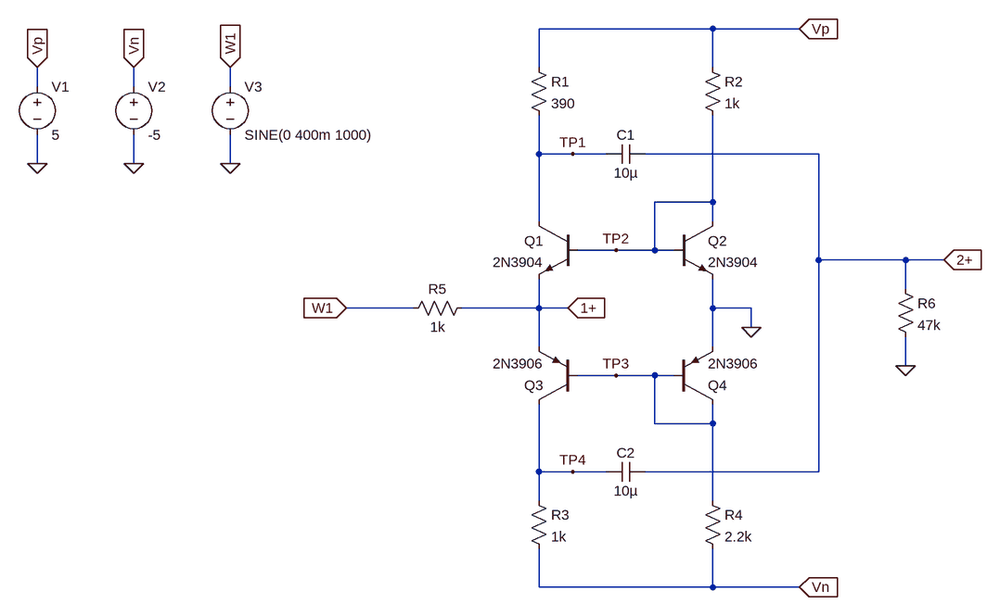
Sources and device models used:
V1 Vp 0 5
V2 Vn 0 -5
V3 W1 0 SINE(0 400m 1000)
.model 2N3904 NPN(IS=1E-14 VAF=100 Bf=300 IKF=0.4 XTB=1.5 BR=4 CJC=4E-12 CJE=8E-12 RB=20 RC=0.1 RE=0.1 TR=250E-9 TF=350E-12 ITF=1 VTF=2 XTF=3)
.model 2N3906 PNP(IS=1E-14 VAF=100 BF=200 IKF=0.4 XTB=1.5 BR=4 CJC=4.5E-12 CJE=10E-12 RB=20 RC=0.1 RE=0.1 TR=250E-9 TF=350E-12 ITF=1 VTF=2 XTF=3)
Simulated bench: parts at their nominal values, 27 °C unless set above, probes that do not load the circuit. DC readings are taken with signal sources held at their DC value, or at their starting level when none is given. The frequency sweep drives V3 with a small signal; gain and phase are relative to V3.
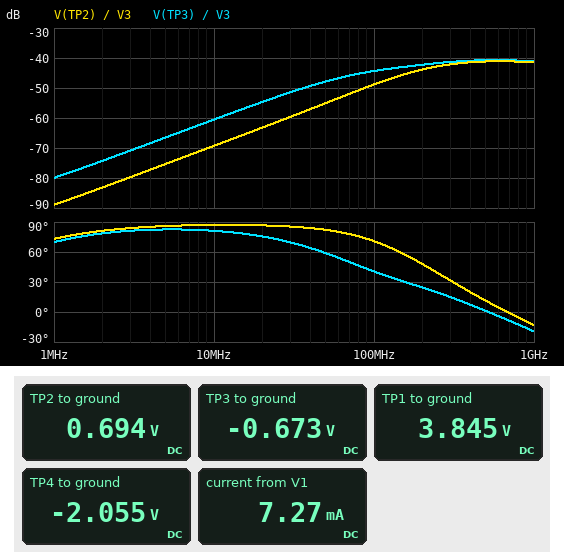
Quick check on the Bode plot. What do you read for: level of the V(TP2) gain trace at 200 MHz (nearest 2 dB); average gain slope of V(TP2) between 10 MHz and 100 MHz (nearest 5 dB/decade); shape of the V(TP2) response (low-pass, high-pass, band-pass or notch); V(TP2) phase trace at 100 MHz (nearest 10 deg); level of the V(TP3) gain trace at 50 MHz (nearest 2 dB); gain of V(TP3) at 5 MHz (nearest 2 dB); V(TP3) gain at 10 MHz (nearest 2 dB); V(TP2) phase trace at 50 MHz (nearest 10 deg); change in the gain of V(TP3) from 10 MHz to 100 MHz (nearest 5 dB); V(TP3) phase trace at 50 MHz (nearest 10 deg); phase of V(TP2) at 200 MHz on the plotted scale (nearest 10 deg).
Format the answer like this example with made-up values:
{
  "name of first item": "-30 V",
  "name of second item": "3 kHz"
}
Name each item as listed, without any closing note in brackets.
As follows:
{
  "level of the V(TP2) gain trace at 200 MHz": "-44 dB",
  "average gain slope of V(TP2) between 10 MHz and 100 MHz": "20 dB/decade",
  "shape of the V(TP2) response": "high-pass",
  "V(TP2) phase trace at 100 MHz": "70 deg",
  "level of the V(TP3) gain trace at 50 MHz": "-48 dB",
  "gain of V(TP3) at 5 MHz": "-66 dB",
  "V(TP3) gain at 10 MHz": "-60 dB",
  "V(TP2) phase trace at 50 MHz": "80 deg",
  "change in the gain of V(TP3) from 10 MHz to 100 MHz": "15 dB",
  "V(TP3) phase trace at 50 MHz": "60 deg",
  "phase of V(TP2) at 200 MHz on the plotted scale": "50 deg"
}
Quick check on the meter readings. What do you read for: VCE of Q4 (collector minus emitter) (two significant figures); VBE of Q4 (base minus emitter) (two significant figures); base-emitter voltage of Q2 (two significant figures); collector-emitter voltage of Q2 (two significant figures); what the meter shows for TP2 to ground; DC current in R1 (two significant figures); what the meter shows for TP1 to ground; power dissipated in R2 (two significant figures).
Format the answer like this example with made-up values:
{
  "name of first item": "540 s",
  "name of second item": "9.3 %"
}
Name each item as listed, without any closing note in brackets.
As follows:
{
  "VCE of Q4 (collector minus emitter)": "-670 mV",
  "VBE of Q4 (base minus emitter)": "-670 mV",
  "base-emitter voltage of Q2": "690 mV",
  "collector-emitter voltage of Q2": "690 mV",
  "what the meter shows for TP2 to ground": "0.694 V",
  "DC current in R1": "3.0 mA",
  "what the meter shows for TP1 to ground": "3.845 V",
  "power dissipated in R2": "19 mW"
}
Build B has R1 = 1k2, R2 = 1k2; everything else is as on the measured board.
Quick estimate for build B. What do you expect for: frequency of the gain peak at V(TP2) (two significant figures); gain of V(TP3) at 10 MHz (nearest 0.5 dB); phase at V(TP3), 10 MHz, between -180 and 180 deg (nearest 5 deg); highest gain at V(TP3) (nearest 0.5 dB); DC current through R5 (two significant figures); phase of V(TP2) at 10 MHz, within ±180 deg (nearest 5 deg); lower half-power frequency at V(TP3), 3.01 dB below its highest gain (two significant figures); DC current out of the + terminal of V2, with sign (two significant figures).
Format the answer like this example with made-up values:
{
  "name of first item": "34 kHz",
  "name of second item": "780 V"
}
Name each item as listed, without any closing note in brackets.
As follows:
{
  "frequency of the gain peak at V(TP2)": "670 MHz",
  "gain of V(TP3) at 10 MHz": "-56.0 dB",
  "phase at V(TP3), 10 MHz, between -180 and 180 deg": "75 deg",
  "highest gain at V(TP3)": "-40.5 dB",
  "DC current through R5": "7.9 µA",
  "phase of V(TP2) at 10 MHz, within ±180 deg": "80 deg",
  "lower half-power frequency at V(TP3), 3.01 dB below its highest gain": "89 MHz",
  "DC current out of the + terminal of V2, with sign": "-4.6 mA"
}
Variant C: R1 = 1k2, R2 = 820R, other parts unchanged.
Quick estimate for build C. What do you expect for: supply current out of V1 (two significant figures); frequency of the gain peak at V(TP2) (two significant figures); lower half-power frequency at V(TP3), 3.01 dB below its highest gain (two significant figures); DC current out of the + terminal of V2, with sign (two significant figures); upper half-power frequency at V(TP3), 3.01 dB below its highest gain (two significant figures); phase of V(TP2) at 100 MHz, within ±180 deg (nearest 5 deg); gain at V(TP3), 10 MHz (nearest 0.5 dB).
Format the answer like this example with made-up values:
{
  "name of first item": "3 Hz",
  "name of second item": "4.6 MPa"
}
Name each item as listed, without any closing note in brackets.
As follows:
{
  "supply current out of V1": "8.5 mA",
  "frequency of the gain peak at V(TP2)": "720 MHz",
  "lower half-power frequency at V(TP3), 3.01 dB below its highest gain": "100 MHz",
  "DC current out of the + terminal of V2, with sign": "-5.2 mA",
  "upper half-power frequency at V(TP3), 3.01 dB below its highest gain": "2.3 GHz",
  "phase of V(TP2) at 100 MHz, within ±180 deg": "50 deg",
  "gain at V(TP3), 10 MHz": "-55.5 dB"
}
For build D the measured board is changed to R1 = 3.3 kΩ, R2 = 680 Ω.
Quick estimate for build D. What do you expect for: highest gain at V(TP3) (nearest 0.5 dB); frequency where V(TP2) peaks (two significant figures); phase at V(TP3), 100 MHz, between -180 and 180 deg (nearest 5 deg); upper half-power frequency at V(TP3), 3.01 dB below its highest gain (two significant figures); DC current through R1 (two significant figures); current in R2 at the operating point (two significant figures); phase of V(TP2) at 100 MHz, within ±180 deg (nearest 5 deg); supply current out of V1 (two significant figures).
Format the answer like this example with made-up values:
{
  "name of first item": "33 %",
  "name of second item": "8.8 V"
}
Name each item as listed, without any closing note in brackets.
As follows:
{
  "highest gain at V(TP3)": "-40.5 dB",
  "frequency where V(TP2) peaks": "830 MHz",
  "phase at V(TP3), 100 MHz, between -180 and 180 deg": "50 deg",
  "upper half-power frequency at V(TP3), 3.01 dB below its highest gain": "2.3 GHz",
  "DC current through R1": "1.5 mA",
  "current in R2 at the operating point": "6.3 mA",
  "phase of V(TP2) at 100 MHz, within ±180 deg": "10 deg",
  "supply current out of V1": "7.8 mA"
}
